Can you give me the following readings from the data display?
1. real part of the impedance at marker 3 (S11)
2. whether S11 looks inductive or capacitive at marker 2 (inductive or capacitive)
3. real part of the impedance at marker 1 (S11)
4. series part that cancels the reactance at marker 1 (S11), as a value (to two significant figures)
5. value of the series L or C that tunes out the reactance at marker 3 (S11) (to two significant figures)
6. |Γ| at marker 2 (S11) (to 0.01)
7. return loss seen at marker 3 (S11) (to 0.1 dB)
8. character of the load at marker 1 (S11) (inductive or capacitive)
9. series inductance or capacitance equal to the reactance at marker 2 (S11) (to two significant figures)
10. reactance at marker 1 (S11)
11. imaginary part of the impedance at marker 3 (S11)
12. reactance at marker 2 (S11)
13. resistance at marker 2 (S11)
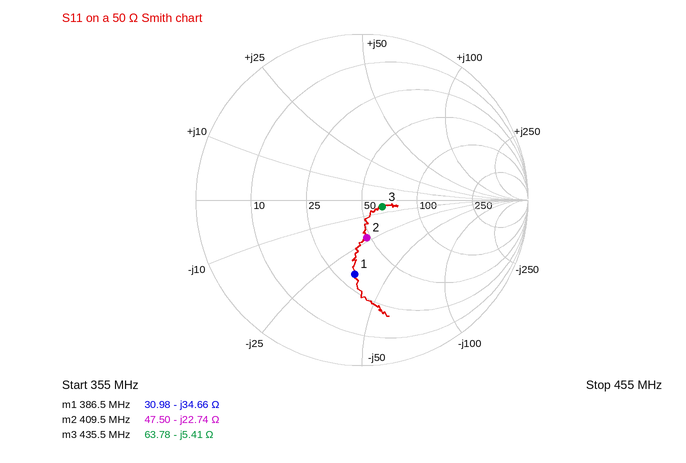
63.78 Ω
capacitive
30.98 Ω
14 nH
2.0 nH
0.23
17.7 dB
capacitive
17 pF
-34.66 Ω
-5.41 Ω
-22.74 Ω
47.50 Ω
